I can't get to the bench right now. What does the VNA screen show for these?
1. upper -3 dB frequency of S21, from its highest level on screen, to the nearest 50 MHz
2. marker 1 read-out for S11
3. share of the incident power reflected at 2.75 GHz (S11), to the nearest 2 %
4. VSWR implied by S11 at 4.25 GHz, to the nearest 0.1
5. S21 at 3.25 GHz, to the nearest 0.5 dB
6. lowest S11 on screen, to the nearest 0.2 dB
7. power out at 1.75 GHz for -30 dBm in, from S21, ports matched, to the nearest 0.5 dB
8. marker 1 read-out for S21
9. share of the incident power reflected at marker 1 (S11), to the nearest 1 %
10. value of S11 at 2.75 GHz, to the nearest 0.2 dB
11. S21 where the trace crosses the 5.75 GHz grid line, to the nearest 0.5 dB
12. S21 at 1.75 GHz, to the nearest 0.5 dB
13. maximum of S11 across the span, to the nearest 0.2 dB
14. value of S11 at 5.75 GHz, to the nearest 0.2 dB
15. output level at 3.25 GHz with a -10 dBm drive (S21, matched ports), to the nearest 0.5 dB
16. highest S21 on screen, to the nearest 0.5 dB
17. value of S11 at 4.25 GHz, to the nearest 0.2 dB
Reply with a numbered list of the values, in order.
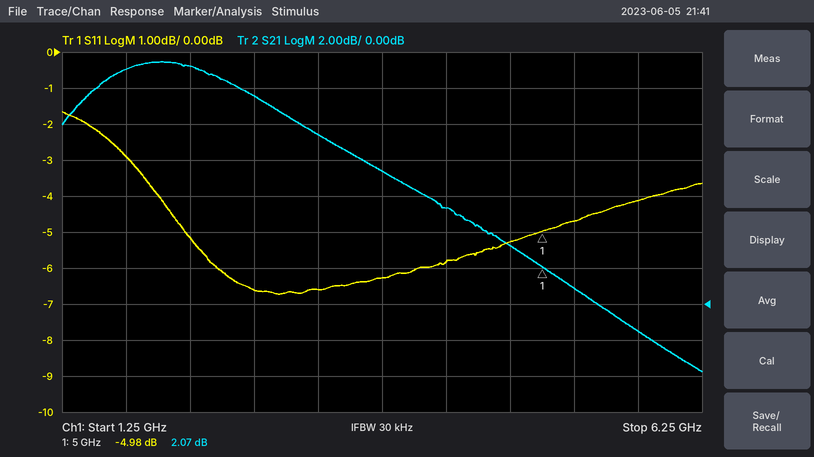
1. 3.00 GHz
2. -4.98 dB
3. 22 %
4. 3.1
5. 9.5 dB
6. -6.8 dB
7. -17.0 dBm
8. 2.07 dB
9. 32 %
10. -6.6 dB
11. -1.5 dB
12. 13.0 dB
13. -1.6 dB
14. -4.2 dB
15. -0.5 dBm
16. 13.5 dB
17. -5.8 dB
